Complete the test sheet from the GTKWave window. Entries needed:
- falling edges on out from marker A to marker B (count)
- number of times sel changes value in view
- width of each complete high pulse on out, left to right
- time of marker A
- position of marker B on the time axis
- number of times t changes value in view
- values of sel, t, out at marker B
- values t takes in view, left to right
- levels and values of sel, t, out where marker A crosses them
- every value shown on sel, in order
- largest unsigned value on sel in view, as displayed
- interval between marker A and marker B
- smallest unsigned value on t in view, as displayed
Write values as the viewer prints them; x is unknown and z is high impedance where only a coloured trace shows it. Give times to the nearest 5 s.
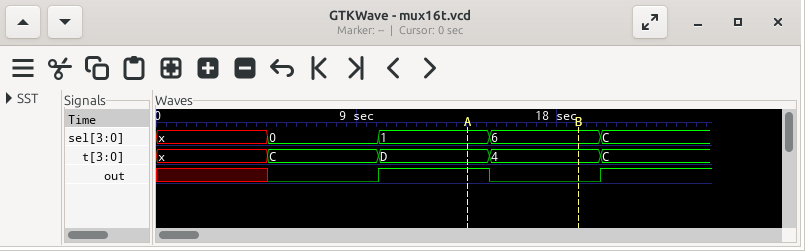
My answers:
1
4
5 s
15 s
20 s
4
sel=6, t=4, out=0
x, C, D, 4, C
sel=1, t=D, out=1
x, 0, 1, 6, C
C
5 s
4
